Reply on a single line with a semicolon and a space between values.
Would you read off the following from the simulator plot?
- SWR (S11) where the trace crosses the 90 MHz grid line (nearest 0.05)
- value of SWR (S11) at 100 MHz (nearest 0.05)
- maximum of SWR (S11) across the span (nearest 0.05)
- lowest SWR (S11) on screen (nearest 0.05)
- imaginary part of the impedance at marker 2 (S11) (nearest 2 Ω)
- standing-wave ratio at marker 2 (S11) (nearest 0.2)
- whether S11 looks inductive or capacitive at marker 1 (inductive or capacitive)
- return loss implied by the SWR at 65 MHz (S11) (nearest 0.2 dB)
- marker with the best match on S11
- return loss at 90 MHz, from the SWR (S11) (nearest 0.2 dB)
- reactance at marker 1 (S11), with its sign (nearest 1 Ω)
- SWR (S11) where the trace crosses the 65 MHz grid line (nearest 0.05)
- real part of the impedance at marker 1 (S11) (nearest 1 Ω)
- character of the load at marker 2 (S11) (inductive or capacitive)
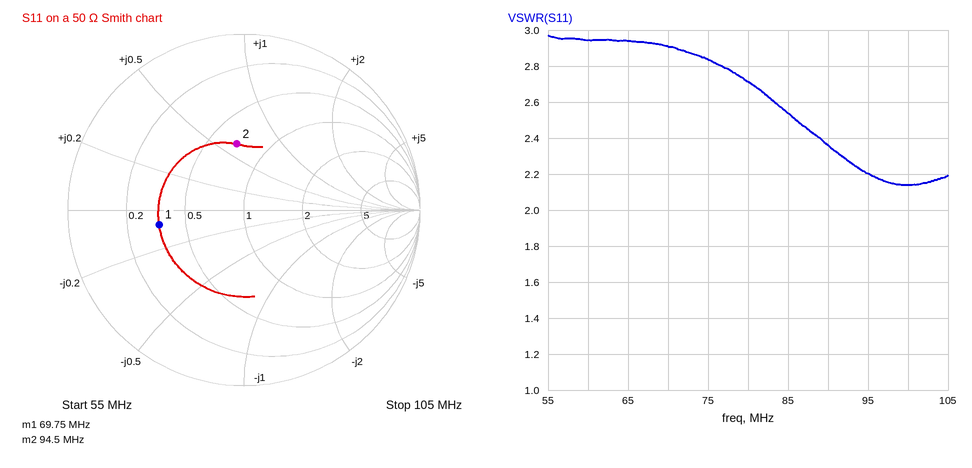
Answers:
2.35; 2.15; 2.95; 2.15; +30 Ω; 2.2; capacitive; 6.2 dB; marker 2; 7.8 dB; -4 Ω; 2.95; 17 Ω; inductive
